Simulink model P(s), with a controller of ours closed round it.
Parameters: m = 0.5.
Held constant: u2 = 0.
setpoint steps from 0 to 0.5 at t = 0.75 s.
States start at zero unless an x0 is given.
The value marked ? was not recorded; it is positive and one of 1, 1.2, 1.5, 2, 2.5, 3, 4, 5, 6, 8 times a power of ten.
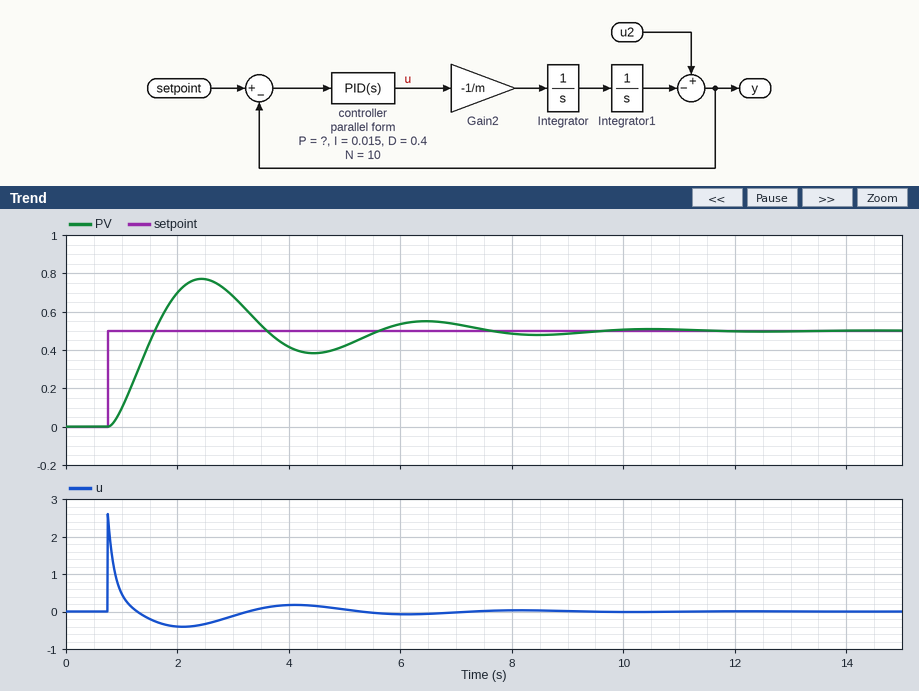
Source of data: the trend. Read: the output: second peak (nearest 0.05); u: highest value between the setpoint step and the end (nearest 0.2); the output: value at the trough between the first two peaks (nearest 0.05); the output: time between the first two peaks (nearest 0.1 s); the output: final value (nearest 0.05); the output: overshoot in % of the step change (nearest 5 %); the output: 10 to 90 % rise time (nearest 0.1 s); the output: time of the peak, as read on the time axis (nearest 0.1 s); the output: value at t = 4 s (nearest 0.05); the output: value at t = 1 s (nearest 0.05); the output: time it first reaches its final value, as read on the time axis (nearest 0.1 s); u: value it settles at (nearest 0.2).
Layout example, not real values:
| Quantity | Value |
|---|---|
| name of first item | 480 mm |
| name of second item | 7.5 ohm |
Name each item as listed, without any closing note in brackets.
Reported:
| Quantity | Value |
|---|---|
| the output: second peak | 0.55 |
| u: highest value between the setpoint step and the end | 2.6 |
| the output: value at the trough between the first two peaks | 0.40 |
| the output: time between the first two peaks | 4.0 s |
| the output: final value | 0.50 |
| the output: overshoot in % of the step change | 55 % |
| the output: 10 to 90 % rise time | 0.6 s |
| the output: time of the peak, as read on the time axis | 2.4 s |
| the output: value at t = 4 s | 0.40 |
| the output: value at t = 1 s | 0.10 |
| the output: time it first reaches its final value, as read on the time axis | 1.6 s |
| u: value it settles at | 0.0 |
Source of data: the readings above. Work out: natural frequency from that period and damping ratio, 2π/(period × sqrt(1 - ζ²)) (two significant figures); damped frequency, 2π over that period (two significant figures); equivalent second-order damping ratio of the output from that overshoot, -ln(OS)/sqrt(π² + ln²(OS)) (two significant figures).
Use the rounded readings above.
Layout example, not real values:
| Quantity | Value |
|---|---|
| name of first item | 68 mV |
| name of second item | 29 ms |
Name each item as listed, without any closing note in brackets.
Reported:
| Quantity | Value |
|---|---|
| natural frequency from that period and damping ratio, 2π/(period × sqrt(1 - ζ²)) | 1.6 rad/s |
| damped frequency, 2π over that period | 1.6 rad/s |
| equivalent second-order damping ratio of the output from that overshoot, -ln(OS)/sqrt(π² + ln²(OS)) | 0.19 |
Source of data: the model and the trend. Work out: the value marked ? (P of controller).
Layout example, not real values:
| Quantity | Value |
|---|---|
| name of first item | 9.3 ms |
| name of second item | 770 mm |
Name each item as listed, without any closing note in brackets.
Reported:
| Quantity | Value |
|---|---|
| the value marked ? | 1.2 |
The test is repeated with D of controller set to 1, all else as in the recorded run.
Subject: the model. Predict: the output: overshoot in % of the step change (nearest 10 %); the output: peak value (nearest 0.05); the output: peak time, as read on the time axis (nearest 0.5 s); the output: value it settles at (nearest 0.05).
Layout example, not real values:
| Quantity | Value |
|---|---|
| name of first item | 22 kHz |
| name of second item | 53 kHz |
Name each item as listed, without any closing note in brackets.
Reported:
| Quantity | Value |
|---|---|
| the output: overshoot in % of the step change | 30 % |
| the output: peak value | 0.65 |
| the output: peak time, as read on the time axis | 2.0 s |
| the output: value it settles at | 0.50 |
